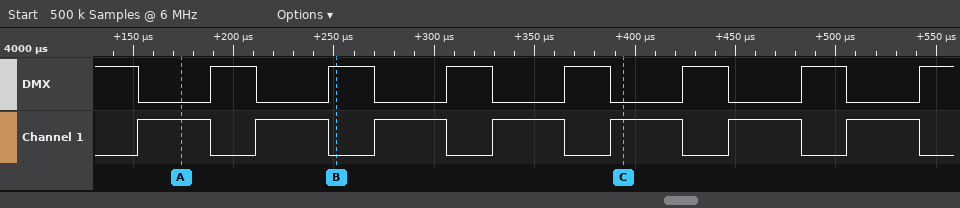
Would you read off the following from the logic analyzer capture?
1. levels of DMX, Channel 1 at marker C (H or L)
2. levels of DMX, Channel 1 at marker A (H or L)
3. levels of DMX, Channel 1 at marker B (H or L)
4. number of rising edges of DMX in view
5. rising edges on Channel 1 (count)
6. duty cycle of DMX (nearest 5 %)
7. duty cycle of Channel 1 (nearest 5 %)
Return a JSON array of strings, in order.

["DMX=L, Channel 1=H", "DMX=L, Channel 1=H", "DMX=H, Channel 1=L", "7", "7", "40 %", "60 %"]
